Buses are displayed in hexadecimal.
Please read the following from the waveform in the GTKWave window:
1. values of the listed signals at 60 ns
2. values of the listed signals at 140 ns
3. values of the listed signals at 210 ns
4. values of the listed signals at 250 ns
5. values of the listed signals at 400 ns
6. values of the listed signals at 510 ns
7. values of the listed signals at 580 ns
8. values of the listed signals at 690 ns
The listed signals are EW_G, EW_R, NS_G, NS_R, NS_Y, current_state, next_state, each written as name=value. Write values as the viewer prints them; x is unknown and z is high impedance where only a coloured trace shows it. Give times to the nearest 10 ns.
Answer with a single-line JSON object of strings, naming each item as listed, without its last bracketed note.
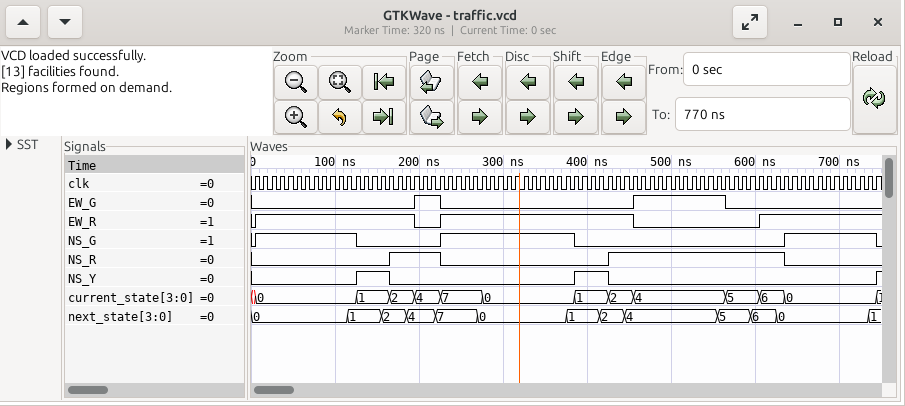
{"values of the listed signals at 60 ns": "EW_G=0, EW_R=1, NS_G=1, NS_R=0, NS_Y=0, current_state=0, next_state=0", "values of the listed signals at 140 ns": "EW_G=0, EW_R=1, NS_G=0, NS_R=0, NS_Y=1, current_state=1, next_state=1", "values of the listed signals at 210 ns": "EW_G=1, EW_R=0, NS_G=0, NS_R=1, NS_Y=0, current_state=4, next_state=4", "values of the listed signals at 250 ns": "EW_G=0, EW_R=1, NS_G=1, NS_R=0, NS_Y=0, current_state=7, next_state=7", "values of the listed signals at 400 ns": "EW_G=0, EW_R=1, NS_G=0, NS_R=0, NS_Y=1, current_state=1, next_state=1", "values of the listed signals at 510 ns": "EW_G=1, EW_R=0, NS_G=0, NS_R=1, NS_Y=0, current_state=4, next_state=4", "values of the listed signals at 580 ns": "EW_G=0, EW_R=0, NS_G=0, NS_R=1, NS_Y=0, current_state=5, next_state=5", "values of the listed signals at 690 ns": "EW_G=0, EW_R=1, NS_G=1, NS_R=0, NS_Y=0, current_state=0, next_state=0"}
